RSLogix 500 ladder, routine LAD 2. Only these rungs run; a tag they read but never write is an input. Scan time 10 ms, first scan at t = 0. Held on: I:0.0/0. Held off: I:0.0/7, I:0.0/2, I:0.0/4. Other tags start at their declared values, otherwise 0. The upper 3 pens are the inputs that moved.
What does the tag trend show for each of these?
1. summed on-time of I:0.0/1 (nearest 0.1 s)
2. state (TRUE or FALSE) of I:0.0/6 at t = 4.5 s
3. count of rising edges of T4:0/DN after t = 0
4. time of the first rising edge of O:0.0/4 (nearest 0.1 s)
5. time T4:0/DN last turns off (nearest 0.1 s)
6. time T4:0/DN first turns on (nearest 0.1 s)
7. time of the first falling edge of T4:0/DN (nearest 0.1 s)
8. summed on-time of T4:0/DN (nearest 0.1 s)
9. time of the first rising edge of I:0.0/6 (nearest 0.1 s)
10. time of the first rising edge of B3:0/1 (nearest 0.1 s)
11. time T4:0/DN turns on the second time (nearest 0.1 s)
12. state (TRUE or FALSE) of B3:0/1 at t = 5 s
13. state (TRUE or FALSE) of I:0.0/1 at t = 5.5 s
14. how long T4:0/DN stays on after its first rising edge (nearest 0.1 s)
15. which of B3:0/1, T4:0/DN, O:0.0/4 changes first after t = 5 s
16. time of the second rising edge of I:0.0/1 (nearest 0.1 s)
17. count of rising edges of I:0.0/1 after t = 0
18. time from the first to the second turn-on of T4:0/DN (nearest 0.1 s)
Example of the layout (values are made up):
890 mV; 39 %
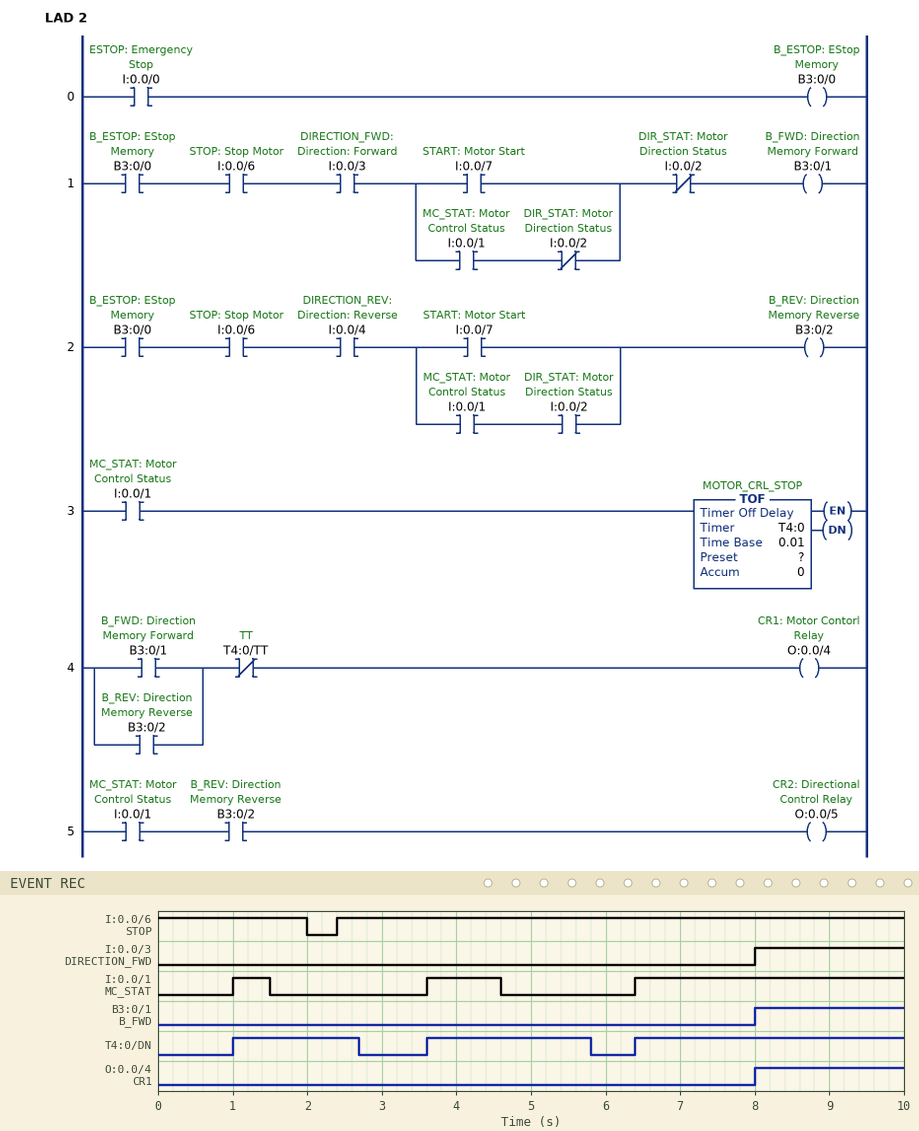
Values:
5.1 s; TRUE; 3; 8.0 s; 5.8 s; 1.0 s; 2.7 s; 7.5 s; 2.4 s; 8.0 s; 3.6 s; FALSE; FALSE; 1.7 s; T4:0/DN; 3.6 s; 3; 2.6 s
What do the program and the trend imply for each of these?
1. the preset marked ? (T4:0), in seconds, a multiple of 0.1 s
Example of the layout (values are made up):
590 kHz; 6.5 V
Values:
1.2 s
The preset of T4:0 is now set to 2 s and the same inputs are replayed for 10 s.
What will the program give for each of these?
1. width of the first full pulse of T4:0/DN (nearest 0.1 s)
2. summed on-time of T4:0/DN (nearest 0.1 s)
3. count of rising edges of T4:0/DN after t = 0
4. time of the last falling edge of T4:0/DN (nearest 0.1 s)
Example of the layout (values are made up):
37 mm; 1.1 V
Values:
2.5 s; 8.9 s; 2; 3.5 s
